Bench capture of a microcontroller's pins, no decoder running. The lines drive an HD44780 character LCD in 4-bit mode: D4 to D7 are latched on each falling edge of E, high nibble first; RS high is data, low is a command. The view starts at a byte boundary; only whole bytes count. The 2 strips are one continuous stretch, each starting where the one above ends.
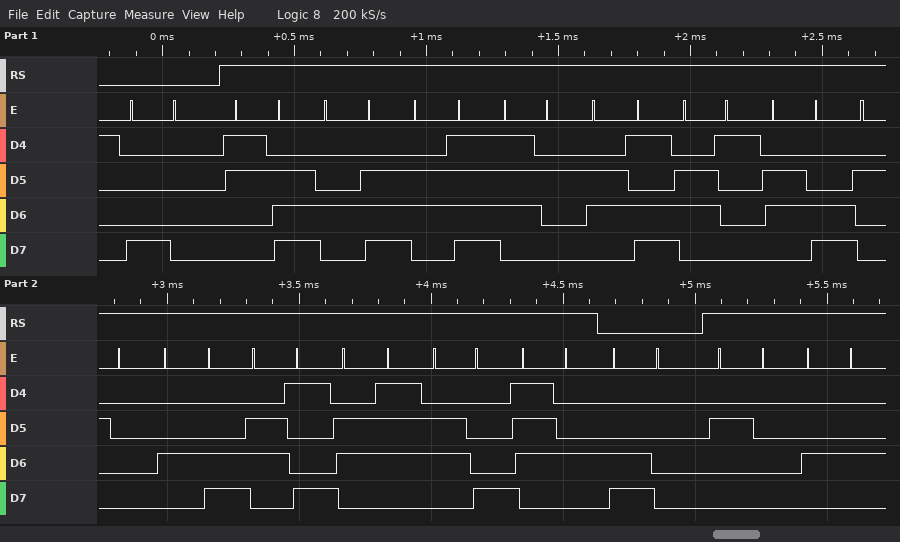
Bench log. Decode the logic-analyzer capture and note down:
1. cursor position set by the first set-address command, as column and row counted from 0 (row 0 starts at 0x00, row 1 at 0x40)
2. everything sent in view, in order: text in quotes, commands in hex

column 0, row 0
0x80 ">Normal Light" 0xC0 " D"
